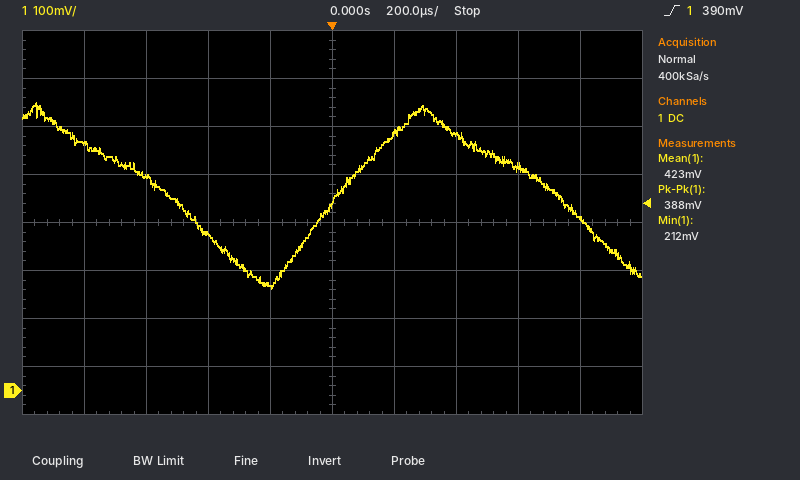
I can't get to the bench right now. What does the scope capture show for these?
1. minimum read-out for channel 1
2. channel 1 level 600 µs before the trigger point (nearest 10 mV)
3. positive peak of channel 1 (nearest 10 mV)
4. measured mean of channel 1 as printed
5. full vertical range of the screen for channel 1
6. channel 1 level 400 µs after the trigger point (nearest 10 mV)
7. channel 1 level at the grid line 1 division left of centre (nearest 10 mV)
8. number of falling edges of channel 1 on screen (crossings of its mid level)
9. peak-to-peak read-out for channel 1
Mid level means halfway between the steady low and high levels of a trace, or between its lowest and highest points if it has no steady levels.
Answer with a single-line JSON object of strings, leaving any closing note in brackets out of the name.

{"minimum read-out for channel 1": "212 mV", "channel 1 level 600 µs before the trigger point": "450 mV", "positive peak of channel 1": "600 mV", "measured mean of channel 1 as printed": "423 mV", "full vertical range of the screen for channel 1": "800 mV", "channel 1 level 400 µs after the trigger point": "530 mV", "channel 1 level at the grid line 1 division left of centre": "220 mV", "number of falling edges of channel 1 on screen": "2", "peak-to-peak read-out for channel 1": "388 mV"}
